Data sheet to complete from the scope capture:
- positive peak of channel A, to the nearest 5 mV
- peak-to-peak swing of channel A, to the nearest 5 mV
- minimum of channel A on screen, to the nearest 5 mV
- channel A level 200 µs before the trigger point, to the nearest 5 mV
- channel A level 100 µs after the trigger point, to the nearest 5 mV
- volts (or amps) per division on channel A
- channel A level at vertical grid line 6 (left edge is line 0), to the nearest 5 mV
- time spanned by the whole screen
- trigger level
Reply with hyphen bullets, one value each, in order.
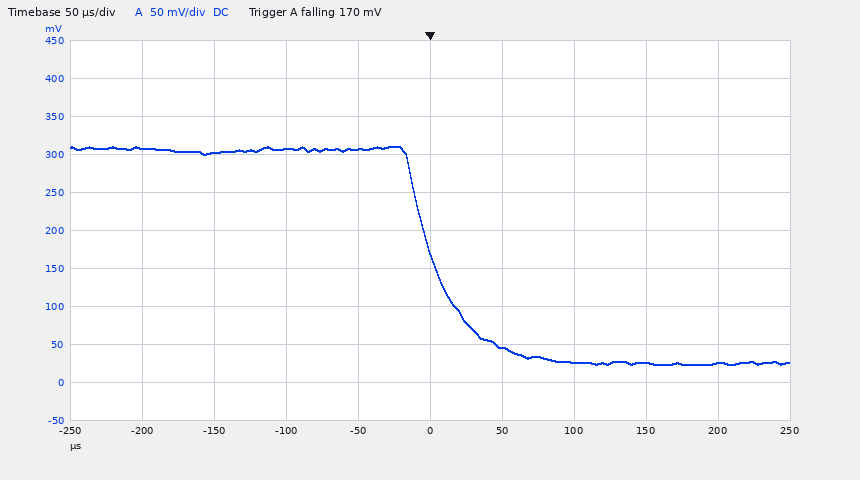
- 310 mV
- 285 mV
- 25 mV
- 310 mV
- 25 mV
- 50 mV
- 45 mV
- 500 µs
- 170 mV
